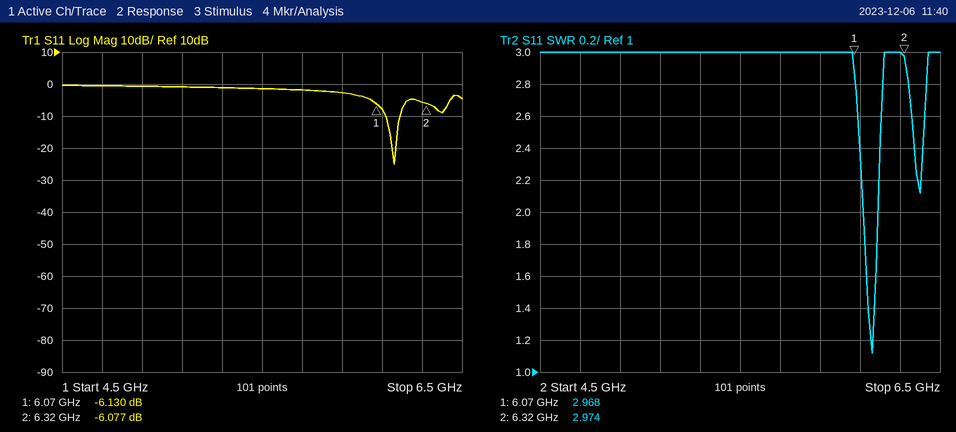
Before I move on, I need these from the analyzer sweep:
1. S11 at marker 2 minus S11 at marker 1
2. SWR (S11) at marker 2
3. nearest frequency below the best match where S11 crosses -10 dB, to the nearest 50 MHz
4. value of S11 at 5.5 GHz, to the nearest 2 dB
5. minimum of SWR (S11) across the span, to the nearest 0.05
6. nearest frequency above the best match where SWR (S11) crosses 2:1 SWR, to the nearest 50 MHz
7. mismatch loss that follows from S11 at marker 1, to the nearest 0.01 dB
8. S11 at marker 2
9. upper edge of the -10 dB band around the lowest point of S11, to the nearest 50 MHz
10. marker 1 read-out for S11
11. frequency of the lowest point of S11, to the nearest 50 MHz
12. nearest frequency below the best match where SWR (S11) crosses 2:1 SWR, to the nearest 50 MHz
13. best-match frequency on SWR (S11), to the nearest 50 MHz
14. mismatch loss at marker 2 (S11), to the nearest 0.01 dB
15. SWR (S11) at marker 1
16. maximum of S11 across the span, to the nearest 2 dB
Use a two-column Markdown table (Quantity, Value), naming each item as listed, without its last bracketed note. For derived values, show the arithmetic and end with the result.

| Quantity | Value |
|---|---|
| S11 at marker 2 minus S11 at marker 1 | -6.077 − (-6.13) = 0.053 dB |
| SWR (S11) at marker 2 | 2.974 |
| nearest frequency below the best match where S11 crosses -10 dB, to the nearest 50 MHz | 6.10 GHz |
| value of S11 at 5.5 GHz, to the nearest 2 dB | -2 dB |
| minimum of SWR (S11) across the span, to the nearest 0.05 | 1.10 |
| nearest frequency above the best match where SWR (S11) crosses 2:1 SWR, to the nearest 50 MHz | 6.20 GHz |
| mismatch loss that follows from S11 at marker 1, to the nearest 0.01 dB | −10 log10(1 − 10^(-6.13/10)) ≈ 1.21 dB |
| S11 at marker 2 | -6.077 dB |
| upper edge of the -10 dB band around the lowest point of S11, to the nearest 50 MHz | 6.20 GHz |
| marker 1 read-out for S11 | -6.130 dB |
| frequency of the lowest point of S11, to the nearest 50 MHz | 6.15 GHz |
| nearest frequency below the best match where SWR (S11) crosses 2:1 SWR, to the nearest 50 MHz | 6.10 GHz |
| best-match frequency on SWR (S11), to the nearest 50 MHz | 6.15 GHz |
| mismatch loss at marker 2 (S11), to the nearest 0.01 dB | −10 log10(1 − 10^(-6.077/10)) ≈ 1.23 dB |
| SWR (S11) at marker 1 | 2.968 |
| maximum of S11 across the span, to the nearest 2 dB | 0 dB |
